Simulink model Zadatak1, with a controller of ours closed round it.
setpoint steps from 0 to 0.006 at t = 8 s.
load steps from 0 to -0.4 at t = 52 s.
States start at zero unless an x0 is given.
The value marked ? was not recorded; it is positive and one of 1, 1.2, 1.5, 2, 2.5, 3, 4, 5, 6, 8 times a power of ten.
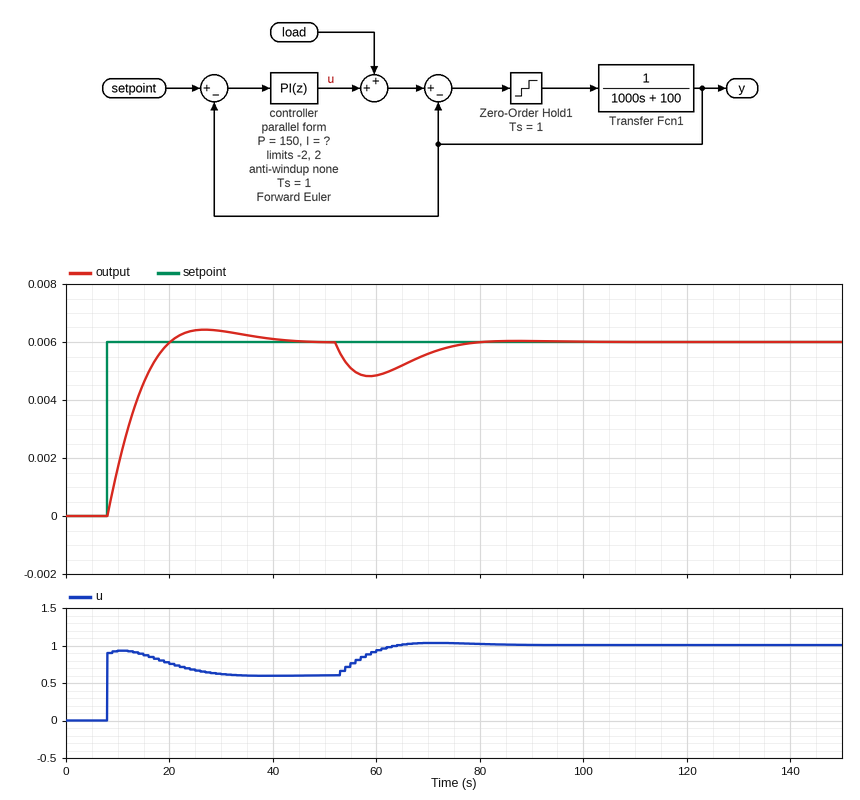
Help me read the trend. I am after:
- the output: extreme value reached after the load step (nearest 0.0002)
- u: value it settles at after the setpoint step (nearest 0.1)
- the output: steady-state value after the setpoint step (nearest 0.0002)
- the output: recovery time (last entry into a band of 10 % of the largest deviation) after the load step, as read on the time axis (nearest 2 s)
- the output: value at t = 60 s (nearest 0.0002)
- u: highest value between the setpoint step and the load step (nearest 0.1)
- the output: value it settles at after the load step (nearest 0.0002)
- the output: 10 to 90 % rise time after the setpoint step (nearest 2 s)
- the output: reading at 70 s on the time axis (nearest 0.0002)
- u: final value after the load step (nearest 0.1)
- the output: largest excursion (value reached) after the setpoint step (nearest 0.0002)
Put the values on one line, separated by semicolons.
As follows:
0.0048; 0.6; 0.0060; 76 s; 0.0048; 0.9; 0.0060; 8 s; 0.0056; 1.0; 0.0064
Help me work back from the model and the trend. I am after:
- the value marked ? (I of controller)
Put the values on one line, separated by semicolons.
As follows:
25
